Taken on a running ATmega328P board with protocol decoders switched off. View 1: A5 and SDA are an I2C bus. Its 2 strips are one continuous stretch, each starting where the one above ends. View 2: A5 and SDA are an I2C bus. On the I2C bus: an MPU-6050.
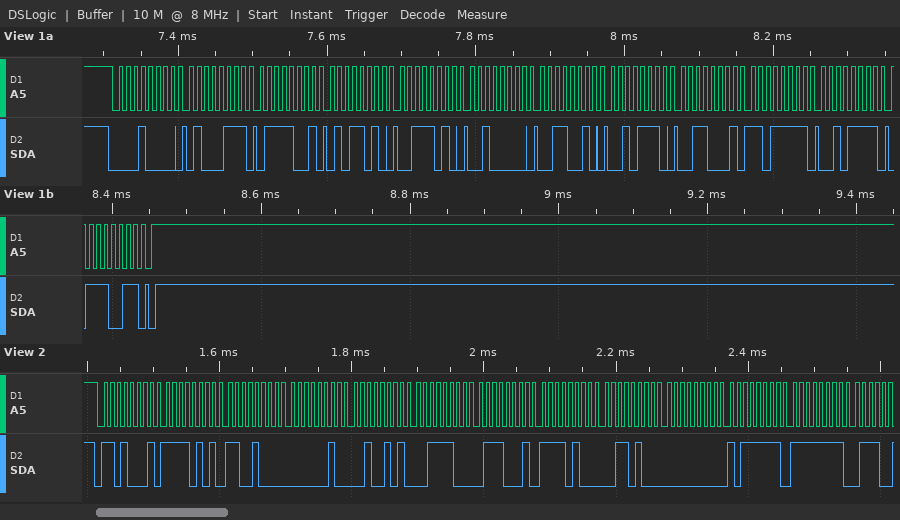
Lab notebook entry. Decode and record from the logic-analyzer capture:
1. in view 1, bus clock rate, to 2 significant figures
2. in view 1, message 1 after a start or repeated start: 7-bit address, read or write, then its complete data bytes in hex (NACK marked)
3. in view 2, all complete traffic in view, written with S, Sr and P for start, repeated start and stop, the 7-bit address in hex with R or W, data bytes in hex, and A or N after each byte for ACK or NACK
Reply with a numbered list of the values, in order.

1. 100 kHz
2. 0x08 write: 47 79 5A 3A 20 32 2E 31 DF 2F 73
3. S 68R A F5 A C8 A 02 A 25 A 3C A 71 A F4 A 34 A 00 A BF A FF A
